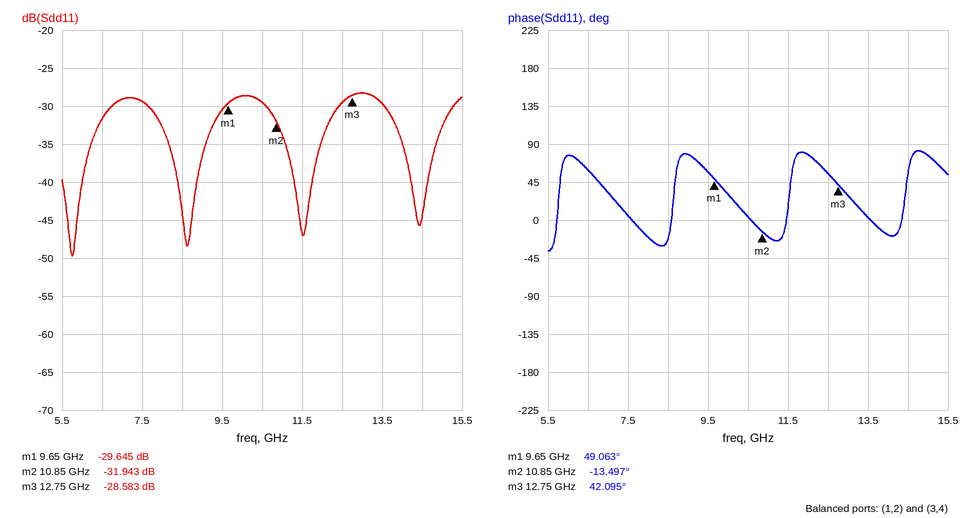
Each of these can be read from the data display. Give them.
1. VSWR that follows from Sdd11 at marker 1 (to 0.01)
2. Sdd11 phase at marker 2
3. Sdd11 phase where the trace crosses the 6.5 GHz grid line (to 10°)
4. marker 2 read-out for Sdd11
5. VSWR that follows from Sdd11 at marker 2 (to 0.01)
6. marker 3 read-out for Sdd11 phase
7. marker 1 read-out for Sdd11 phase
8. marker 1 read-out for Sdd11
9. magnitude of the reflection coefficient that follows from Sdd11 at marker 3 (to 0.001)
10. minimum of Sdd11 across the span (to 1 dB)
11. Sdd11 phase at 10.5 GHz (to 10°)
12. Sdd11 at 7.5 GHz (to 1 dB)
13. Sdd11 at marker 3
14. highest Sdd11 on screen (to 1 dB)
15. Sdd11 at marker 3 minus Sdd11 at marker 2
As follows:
1.07
-13.497°
60°
-31.943 dB
1.05
42.095°
49.063°
-29.645 dB
0.037
-50 dB
0°
-29 dB
-28.583 dB
-28 dB
3.360 dB
